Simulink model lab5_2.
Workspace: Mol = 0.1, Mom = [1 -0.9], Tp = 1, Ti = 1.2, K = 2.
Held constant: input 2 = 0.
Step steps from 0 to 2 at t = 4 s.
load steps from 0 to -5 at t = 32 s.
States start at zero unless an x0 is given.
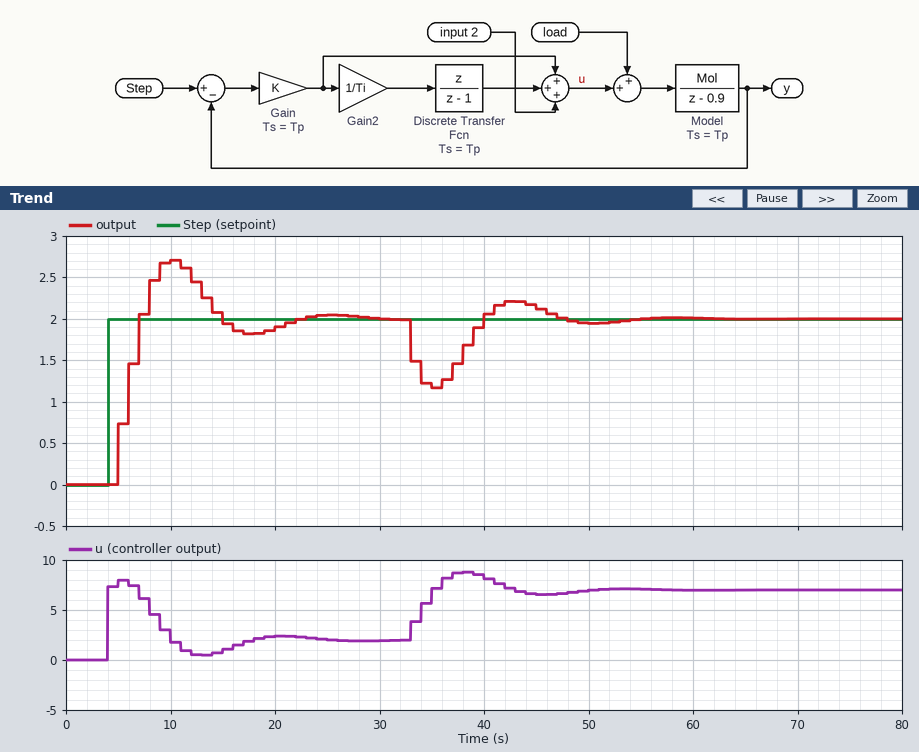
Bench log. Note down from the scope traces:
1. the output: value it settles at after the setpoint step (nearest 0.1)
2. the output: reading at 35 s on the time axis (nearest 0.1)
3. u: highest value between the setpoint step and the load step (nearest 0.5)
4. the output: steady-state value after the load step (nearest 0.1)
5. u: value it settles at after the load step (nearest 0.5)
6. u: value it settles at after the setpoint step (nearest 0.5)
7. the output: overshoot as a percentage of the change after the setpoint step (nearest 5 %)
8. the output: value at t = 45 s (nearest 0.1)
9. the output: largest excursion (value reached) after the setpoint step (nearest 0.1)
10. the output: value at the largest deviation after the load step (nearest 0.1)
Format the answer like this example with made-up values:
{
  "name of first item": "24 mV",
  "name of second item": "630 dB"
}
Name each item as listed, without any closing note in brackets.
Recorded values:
{
  "the output: value it settles at after the setpoint step": "2.0",
  "the output: reading at 35 s on the time axis": "1.2",
  "u: highest value between the setpoint step and the load step": "8.0",
  "the output: steady-state value after the load step": "2.0",
  "u: value it settles at after the load step": "7.0",
  "u: value it settles at after the setpoint step": "2.0",
  "the output: overshoot as a percentage of the change after the setpoint step": "35 %",
  "the output: value at t = 45 s": "2.1",
  "the output: largest excursion (value reached) after the setpoint step": "2.7",
  "the output: value at the largest deviation after the load step": "1.2"
}
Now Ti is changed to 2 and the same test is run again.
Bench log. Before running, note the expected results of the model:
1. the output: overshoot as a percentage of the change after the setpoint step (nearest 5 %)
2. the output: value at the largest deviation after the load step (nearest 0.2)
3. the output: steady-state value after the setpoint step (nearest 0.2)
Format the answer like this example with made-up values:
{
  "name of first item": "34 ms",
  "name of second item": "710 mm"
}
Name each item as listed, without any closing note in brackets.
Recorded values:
{
  "the output: overshoot as a percentage of the change after the setpoint step": "25 %",
  "the output: value at the largest deviation after the load step": "1.0",
  "the output: steady-state value after the setpoint step": "2.0"
}
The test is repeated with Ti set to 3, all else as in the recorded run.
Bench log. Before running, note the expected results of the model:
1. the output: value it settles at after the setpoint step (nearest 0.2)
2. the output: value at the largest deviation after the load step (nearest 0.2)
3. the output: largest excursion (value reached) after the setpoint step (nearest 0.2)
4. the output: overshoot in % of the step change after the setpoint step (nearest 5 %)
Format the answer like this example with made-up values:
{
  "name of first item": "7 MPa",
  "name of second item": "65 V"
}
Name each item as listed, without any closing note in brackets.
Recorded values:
{
  "the output: value it settles at after the setpoint step": "2.0",
  "the output: value at the largest deviation after the load step": "1.0",
  "the output: largest excursion (value reached) after the setpoint step": "2.4",
  "the output: overshoot in % of the step change after the setpoint step": "15 %"
}
